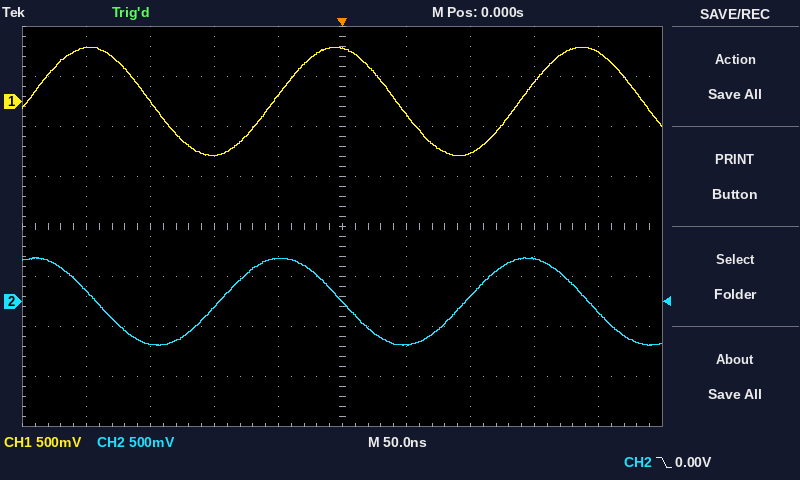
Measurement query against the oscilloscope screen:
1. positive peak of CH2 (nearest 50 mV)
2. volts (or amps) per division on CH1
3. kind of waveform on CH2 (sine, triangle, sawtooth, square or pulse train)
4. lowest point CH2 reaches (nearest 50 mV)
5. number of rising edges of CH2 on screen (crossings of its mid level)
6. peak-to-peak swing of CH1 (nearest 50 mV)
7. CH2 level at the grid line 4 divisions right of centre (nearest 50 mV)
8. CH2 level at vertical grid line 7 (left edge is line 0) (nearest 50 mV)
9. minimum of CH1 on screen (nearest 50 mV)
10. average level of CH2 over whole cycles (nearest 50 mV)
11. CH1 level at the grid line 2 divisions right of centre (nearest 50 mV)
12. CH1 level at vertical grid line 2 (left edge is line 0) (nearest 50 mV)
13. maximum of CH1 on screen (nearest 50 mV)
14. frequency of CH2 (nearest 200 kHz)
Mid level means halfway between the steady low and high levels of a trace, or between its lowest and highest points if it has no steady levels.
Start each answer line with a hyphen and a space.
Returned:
- 450 mV
- 500 mV
- sine
- -450 mV
- 2
- 1.10 V
- -100 mV
- 50 mV
- -550 mV
- 0 mV
- -500 mV
- 0 mV
- 550 mV
- 5.2 MHz
